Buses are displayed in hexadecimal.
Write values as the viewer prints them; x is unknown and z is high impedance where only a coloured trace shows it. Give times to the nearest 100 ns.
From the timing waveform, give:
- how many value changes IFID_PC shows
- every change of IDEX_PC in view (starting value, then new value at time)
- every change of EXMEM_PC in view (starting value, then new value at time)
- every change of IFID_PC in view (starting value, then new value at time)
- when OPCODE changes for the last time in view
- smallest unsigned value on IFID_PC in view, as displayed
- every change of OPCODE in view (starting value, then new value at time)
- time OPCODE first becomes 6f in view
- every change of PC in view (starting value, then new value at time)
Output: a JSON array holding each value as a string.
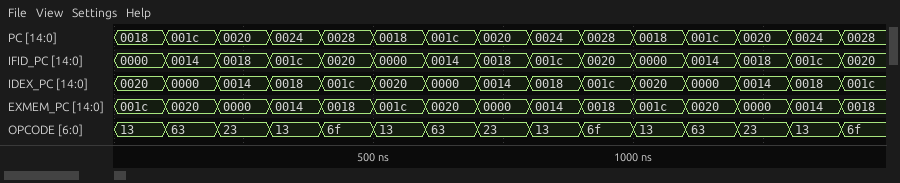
["14", "0020, 0000 at 100 ns, 0014 at 200 ns, 0018 at 300 ns, 001c at 400 ns, 0020 at 500 ns, 0000 at 600 ns, 0014 at 700 ns, 0018 at 800 ns, 001c at 900 ns, 0020 at 1000 ns, 0000 at 1100 ns, 0014 at 1200 ns, 0018 at 1300 ns, 001c at 1400 ns", "001c, 0020 at 100 ns, 0000 at 200 ns, 0014 at 300 ns, 0018 at 400 ns, 001c at 500 ns, 0020 at 600 ns, 0000 at 700 ns, 0014 at 800 ns, 0018 at 900 ns, 001c at 1000 ns, 0020 at 1100 ns, 0000 at 1200 ns, 0014 at 1300 ns, 0018 at 1400 ns", "0000, 0014 at 100 ns, 0018 at 200 ns, 001c at 300 ns, 0020 at 400 ns, 0000 at 500 ns, 0014 at 600 ns, 0018 at 700 ns, 001c at 800 ns, 0020 at 900 ns, 0000 at 1000 ns, 0014 at 1100 ns, 0018 at 1200 ns, 001c at 1300 ns, 0020 at 1400 ns", "1400 ns", "0000", "13, 63 at 100 ns, 23 at 200 ns, 13 at 300 ns, 6f at 400 ns, 13 at 500 ns, 63 at 600 ns, 23 at 700 ns, 13 at 800 ns, 6f at 900 ns, 13 at 1000 ns, 63 at 1100 ns, 23 at 1200 ns, 13 at 1300 ns, 6f at 1400 ns", "400 ns", "0018, 001c at 100 ns, 0020 at 200 ns, 0024 at 300 ns, 0028 at 400 ns, 0018 at 500 ns, 001c at 600 ns, 0020 at 700 ns, 0024 at 800 ns, 0028 at 900 ns, 0018 at 1000 ns, 001c at 1100 ns, 0020 at 1200 ns, 0024 at 1300 ns, 0028 at 1400 ns"]
